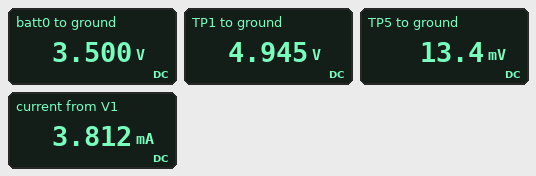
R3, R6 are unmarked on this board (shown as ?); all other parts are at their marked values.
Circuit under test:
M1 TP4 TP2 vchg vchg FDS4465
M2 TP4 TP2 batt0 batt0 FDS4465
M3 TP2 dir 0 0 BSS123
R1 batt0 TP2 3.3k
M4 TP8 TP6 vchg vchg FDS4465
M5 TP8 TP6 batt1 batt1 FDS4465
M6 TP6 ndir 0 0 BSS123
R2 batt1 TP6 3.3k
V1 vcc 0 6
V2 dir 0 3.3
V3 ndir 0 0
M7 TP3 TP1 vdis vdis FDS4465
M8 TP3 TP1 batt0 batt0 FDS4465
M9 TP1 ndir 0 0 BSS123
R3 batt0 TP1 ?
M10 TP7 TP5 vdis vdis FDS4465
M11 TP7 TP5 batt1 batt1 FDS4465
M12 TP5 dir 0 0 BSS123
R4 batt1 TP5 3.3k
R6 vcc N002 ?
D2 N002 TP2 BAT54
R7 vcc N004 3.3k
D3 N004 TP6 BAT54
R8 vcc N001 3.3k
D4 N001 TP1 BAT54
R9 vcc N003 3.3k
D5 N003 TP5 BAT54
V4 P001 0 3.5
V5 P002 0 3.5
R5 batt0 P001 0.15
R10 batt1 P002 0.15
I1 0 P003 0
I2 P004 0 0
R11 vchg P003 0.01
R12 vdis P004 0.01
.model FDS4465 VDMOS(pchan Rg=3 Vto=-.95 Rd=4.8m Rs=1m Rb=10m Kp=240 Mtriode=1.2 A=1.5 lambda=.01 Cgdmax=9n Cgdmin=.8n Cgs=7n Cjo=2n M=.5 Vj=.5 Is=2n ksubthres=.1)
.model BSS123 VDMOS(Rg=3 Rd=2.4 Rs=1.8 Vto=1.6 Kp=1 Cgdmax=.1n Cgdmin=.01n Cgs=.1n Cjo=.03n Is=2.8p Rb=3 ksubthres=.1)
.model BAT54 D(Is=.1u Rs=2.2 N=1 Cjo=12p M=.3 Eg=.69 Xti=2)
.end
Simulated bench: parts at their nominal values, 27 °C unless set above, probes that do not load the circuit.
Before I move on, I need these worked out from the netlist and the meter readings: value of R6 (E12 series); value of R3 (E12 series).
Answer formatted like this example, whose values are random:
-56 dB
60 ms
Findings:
3.9 kΩ
5.6 kΩ
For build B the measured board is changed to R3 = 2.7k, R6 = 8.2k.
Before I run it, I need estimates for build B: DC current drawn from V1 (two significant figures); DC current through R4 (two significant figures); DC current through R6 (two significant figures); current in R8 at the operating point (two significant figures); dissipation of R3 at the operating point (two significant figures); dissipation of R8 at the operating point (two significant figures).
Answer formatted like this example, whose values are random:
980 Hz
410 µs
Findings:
3.2 mA
1.1 mA
700 µA
380 µA
390 µW
480 µW
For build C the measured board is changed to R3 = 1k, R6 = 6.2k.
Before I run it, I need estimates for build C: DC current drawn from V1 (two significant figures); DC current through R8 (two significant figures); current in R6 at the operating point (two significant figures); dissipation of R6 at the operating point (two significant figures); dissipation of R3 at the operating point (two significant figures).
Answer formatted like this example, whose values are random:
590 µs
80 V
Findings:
3.5 mA
530 µA
930 µA
5.3 mW
280 µW
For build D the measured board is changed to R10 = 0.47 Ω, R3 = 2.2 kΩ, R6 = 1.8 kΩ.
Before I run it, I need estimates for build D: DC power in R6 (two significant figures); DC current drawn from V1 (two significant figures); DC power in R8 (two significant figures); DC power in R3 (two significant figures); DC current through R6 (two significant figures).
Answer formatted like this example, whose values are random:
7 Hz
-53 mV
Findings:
18 mW
5.7 mA
570 µW
380 µW
3.2 mA
